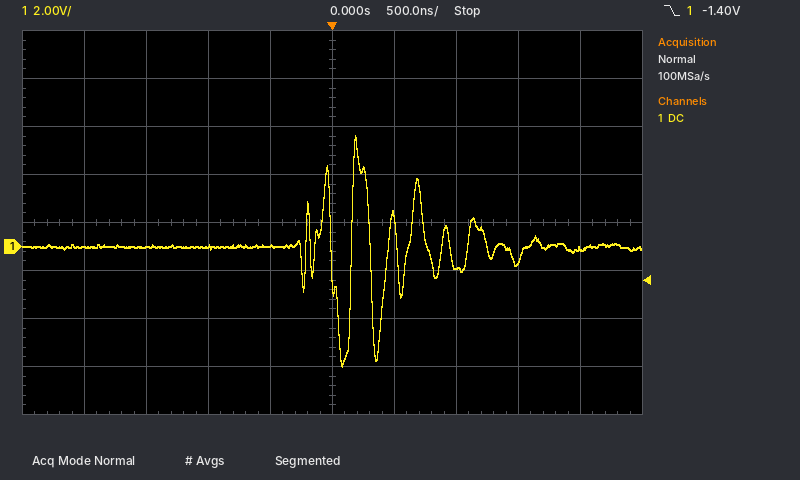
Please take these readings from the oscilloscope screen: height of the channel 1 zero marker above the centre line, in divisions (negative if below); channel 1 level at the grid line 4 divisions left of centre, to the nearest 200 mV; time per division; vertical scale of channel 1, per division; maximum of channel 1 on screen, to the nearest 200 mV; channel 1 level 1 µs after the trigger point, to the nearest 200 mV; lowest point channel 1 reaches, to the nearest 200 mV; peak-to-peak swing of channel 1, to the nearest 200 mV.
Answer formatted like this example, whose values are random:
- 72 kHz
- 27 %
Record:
- -0.5 div
- 0.0 V
- 500 ns
- 2 V
- 4.6 V
- -800 mV
- -5.0 V
- 9.6 V
